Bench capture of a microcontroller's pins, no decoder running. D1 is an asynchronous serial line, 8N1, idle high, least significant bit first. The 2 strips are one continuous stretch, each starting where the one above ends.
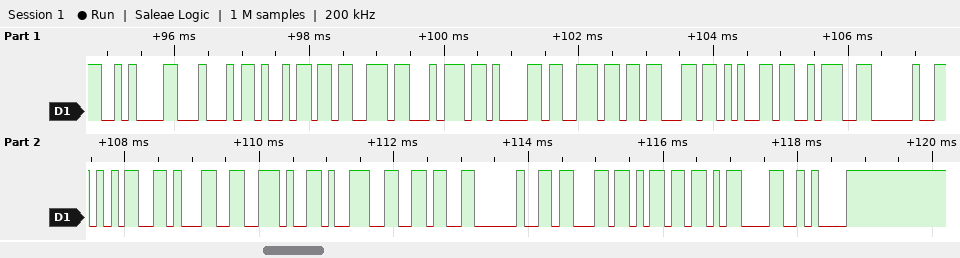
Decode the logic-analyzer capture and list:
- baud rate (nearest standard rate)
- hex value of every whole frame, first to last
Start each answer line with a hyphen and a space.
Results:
- 9600 baud
- 0x0A 0x44 0x69 0x73 0x74 0x61 0x6E 0x63 0x65 0x3A 0x20 0x35 0x31 0x2E 0x39 0x36 0x20 0x63 0x6D 0x0D 0x0A
